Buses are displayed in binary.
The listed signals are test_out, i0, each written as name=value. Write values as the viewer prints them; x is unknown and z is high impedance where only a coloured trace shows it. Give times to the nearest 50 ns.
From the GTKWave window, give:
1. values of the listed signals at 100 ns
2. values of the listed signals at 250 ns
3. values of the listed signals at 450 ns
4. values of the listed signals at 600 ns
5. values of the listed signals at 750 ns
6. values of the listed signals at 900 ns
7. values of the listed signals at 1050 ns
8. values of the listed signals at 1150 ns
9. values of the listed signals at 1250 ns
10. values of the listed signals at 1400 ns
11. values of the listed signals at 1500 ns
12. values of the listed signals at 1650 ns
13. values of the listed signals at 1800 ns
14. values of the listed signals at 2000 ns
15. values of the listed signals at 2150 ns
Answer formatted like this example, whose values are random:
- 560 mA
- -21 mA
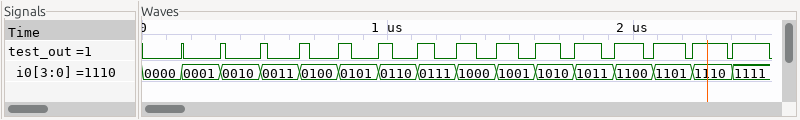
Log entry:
- test_out=0, i0=0000
- test_out=0, i0=0001
- test_out=0, i0=0010
- test_out=0, i0=0011
- test_out=0, i0=0100
- test_out=0, i0=0101
- test_out=0, i0=0110
- test_out=1, i0=0111
- test_out=0, i0=0111
- test_out=0, i0=1000
- test_out=1, i0=1001
- test_out=1, i0=1010
- test_out=1, i0=1011
- test_out=1, i0=1100
- test_out=1, i0=1101
